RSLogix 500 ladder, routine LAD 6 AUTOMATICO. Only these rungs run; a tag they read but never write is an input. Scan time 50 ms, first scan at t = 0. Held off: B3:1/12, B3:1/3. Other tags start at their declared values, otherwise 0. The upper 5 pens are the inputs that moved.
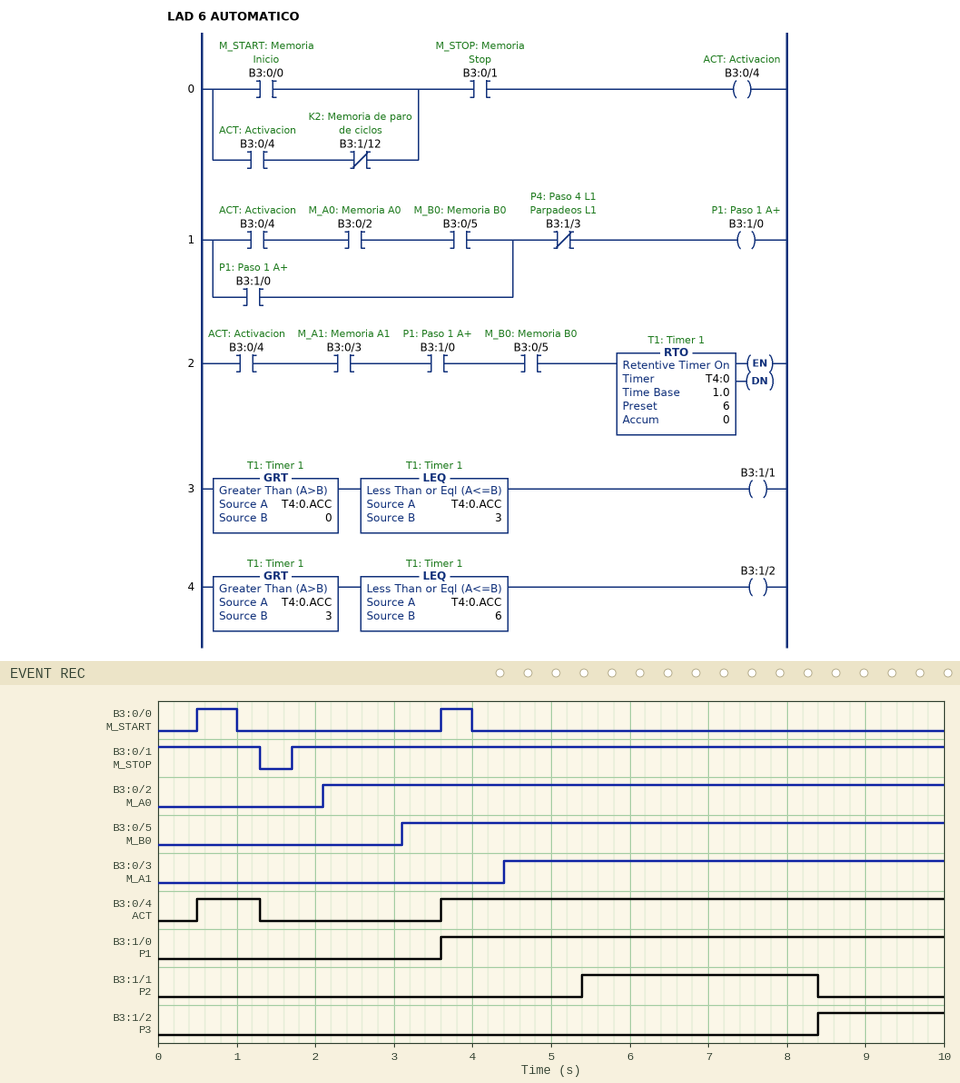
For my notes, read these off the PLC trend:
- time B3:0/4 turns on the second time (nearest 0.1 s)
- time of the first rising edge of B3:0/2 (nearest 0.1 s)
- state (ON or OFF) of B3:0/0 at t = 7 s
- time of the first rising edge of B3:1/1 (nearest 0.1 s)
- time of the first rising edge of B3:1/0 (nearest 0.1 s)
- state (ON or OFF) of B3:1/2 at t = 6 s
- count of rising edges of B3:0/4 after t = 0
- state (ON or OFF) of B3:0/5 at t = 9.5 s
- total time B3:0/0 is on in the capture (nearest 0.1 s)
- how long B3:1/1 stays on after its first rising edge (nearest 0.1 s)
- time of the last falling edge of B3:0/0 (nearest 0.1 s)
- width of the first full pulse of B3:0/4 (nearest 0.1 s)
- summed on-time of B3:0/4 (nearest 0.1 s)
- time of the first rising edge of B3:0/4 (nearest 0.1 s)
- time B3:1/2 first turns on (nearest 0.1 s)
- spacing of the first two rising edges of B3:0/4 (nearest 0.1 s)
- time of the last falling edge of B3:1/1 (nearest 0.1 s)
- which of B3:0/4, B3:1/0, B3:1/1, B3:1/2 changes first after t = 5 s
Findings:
3.6 s
2.1 s
OFF
5.4 s
3.6 s
OFF
2
ON
0.9 s
3.0 s
4.0 s
0.8 s
7.2 s
0.5 s
8.4 s
3.1 s
8.4 s
B3:1/1
